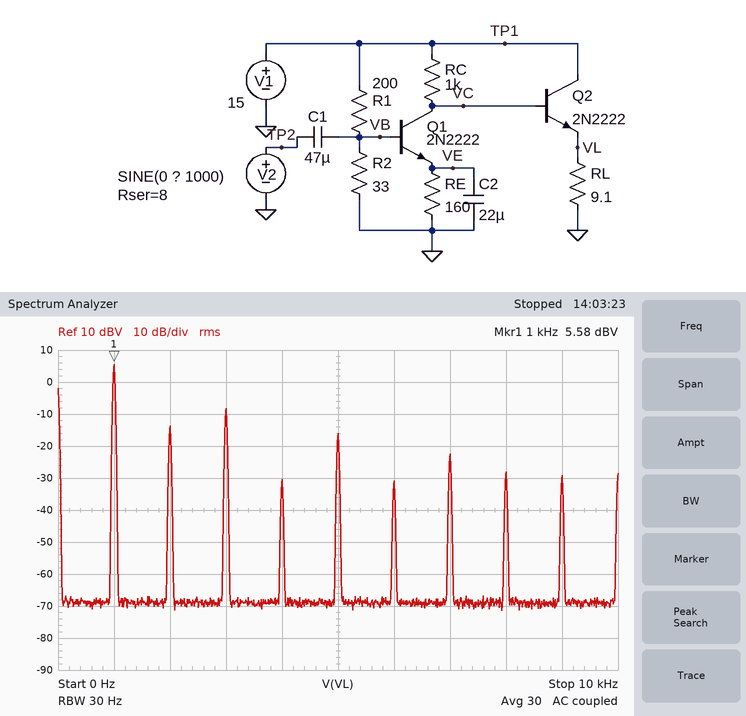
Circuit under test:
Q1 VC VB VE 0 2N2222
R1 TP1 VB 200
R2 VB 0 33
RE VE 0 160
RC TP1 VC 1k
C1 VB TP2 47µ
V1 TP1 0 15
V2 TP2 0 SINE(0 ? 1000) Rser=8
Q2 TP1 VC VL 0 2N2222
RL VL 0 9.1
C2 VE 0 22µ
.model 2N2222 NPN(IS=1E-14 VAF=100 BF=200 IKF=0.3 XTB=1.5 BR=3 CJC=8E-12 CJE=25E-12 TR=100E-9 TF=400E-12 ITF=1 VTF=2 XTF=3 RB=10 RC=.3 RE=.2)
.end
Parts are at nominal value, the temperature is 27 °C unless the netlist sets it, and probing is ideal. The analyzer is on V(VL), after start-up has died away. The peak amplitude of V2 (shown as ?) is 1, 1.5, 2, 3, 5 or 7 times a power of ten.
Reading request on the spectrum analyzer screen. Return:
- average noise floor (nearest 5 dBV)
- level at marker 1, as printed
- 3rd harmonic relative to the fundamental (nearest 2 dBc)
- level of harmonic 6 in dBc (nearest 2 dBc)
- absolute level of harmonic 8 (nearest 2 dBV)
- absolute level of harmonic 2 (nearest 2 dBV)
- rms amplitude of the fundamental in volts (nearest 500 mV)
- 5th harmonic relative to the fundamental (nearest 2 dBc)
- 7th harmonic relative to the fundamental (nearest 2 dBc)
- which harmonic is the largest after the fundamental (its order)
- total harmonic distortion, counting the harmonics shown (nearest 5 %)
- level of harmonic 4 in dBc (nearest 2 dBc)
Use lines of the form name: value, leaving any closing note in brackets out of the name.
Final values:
average noise floor: -70 dBV
level at marker 1, as printed: 5.58 dBV
3rd harmonic relative to the fundamental: -14 dBc
level of harmonic 6 in dBc: -36 dBc
absolute level of harmonic 8: -28 dBV
absolute level of harmonic 2: -14 dBV
rms amplitude of the fundamental in volts: 2.0 V
5th harmonic relative to the fundamental: -22 dBc
7th harmonic relative to the fundamental: -28 dBc
which harmonic is the largest after the fundamental: 3
total harmonic distortion, counting the harmonics shown: 25 %
level of harmonic 4 in dBc: -36 dBc
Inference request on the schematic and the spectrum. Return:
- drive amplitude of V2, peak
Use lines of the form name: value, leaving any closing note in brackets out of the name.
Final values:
drive amplitude of V2, peak: 100 mV
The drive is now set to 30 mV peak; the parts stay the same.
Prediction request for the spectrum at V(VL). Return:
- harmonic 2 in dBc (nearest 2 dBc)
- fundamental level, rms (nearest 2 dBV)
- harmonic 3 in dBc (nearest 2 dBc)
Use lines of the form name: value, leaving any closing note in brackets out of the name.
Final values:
harmonic 2 in dBc: -22 dBc
fundamental level, rms: -2 dBV
harmonic 3 in dBc: -46 dBc
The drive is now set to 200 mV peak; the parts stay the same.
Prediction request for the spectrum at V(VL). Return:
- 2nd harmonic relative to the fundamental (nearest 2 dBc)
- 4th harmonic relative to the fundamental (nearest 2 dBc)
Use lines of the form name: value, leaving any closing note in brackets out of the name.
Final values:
2nd harmonic relative to the fundamental: -24 dBc
4th harmonic relative to the fundamental: -30 dBc
